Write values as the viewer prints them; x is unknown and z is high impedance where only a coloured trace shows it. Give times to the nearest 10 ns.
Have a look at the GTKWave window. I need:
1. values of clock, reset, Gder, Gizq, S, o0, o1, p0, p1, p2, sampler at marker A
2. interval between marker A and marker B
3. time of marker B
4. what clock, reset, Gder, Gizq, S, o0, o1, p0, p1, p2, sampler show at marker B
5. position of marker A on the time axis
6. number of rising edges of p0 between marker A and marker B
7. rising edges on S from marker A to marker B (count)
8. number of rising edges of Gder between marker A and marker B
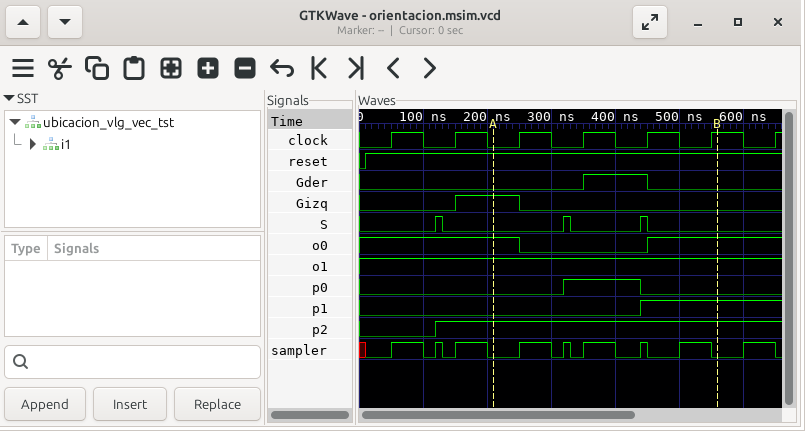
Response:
clock=0, reset=1, Gder=0, Gizq=1, S=0, o0=1, o1=1, p0=0, p1=0, p2=1, sampler=0
350 ns
560 ns
clock=1, reset=1, Gder=0, Gizq=0, S=0, o0=1, o1=1, p0=0, p1=1, p2=1, sampler=0
210 ns
1
2
1
